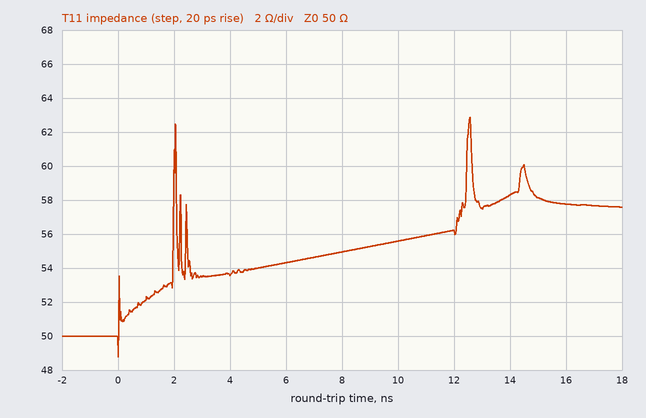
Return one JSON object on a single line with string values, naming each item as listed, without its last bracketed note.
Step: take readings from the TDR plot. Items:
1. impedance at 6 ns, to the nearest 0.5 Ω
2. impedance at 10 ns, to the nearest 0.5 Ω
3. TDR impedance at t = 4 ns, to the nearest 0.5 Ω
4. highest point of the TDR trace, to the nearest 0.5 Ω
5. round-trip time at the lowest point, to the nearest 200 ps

{"impedance at 6 ns, to the nearest 0.5 Ω": "54.5 Ω", "impedance at 10 ns, to the nearest 0.5 Ω": "55.5 Ω", "TDR impedance at t = 4 ns, to the nearest 0.5 Ω": "53.5 Ω", "highest point of the TDR trace, to the nearest 0.5 Ω": "63.0 Ω", "round-trip time at the lowest point, to the nearest 200 ps": "0.0 ns"}
